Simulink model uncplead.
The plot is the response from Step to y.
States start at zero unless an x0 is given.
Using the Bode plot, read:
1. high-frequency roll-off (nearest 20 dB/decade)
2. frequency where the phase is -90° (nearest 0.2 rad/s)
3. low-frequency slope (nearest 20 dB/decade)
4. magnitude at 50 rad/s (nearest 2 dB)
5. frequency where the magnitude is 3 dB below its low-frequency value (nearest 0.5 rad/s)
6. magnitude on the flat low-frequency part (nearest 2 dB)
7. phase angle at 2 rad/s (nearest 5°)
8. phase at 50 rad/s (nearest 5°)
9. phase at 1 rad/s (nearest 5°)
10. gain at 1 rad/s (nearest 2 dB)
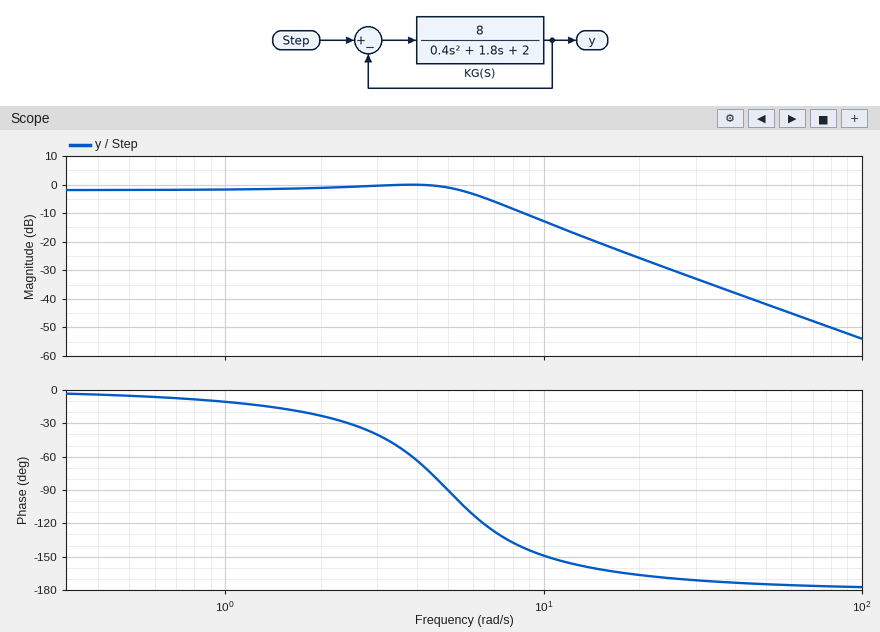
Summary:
-40 dB/decade
5.0 rad/s
0 dB/decade
-42 dB
6.5 rad/s
-2 dB
-25°
-175°
-10°
-2 dB
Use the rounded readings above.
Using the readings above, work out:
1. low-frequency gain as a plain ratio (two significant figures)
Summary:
0.79
